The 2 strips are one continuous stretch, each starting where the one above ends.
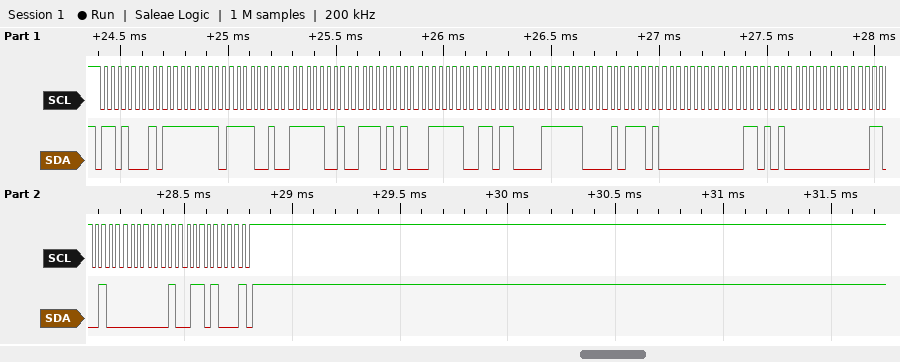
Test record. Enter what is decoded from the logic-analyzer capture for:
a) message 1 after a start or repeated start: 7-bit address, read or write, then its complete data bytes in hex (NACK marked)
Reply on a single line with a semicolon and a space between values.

0x68 read: FF F2 F9 75 3E D8 FC 5D 00 35 00 32 01 68 NACK
